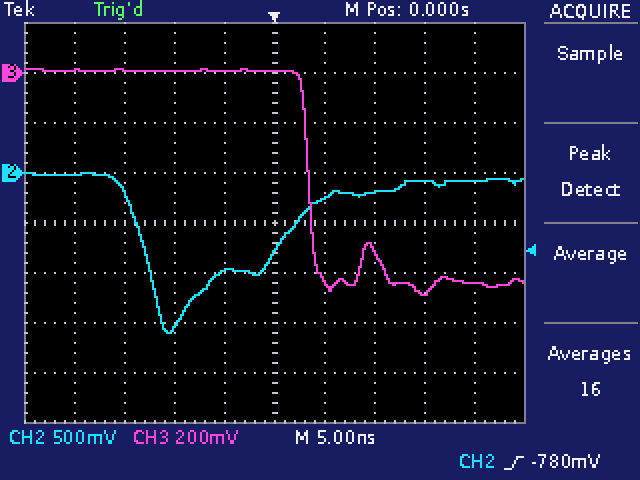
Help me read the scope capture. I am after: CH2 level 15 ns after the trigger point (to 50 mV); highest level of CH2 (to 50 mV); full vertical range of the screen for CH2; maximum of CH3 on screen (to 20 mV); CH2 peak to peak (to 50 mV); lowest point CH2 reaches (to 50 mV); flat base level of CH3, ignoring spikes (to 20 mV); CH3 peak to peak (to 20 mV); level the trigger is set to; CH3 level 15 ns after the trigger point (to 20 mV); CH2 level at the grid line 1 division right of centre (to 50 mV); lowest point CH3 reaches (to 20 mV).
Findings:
-100 mV
0 mV
4 V
20 mV
1.60 V
-1.60 V
-840 mV
900 mV
-780 mV
-880 mV
-250 mV
-880 mV
